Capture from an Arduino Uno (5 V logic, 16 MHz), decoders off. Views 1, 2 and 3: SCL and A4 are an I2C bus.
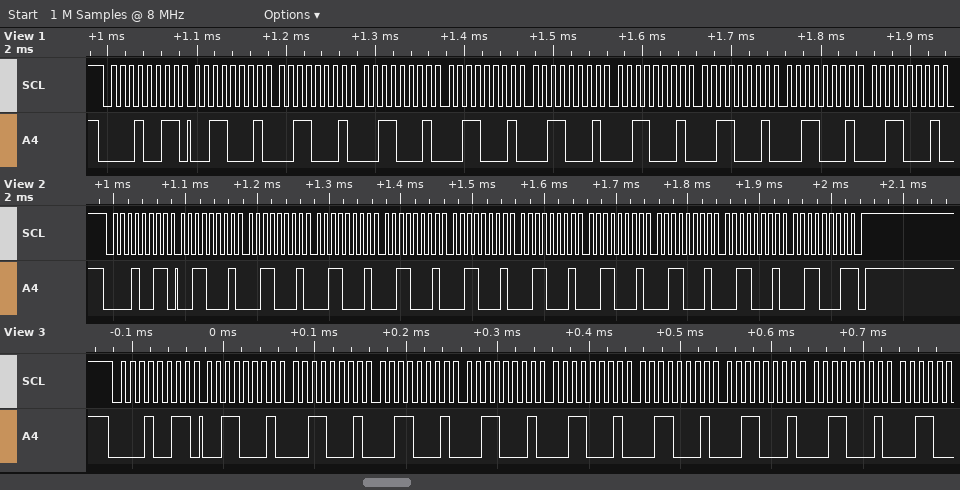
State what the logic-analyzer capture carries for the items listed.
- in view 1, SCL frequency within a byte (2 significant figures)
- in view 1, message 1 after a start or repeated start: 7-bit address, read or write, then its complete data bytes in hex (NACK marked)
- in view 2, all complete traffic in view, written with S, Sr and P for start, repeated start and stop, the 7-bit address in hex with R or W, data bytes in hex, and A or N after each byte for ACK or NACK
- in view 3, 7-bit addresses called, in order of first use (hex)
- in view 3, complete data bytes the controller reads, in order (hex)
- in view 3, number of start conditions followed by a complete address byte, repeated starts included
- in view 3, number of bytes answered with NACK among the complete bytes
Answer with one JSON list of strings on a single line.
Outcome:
["100 kHz", "0x09 read: 31 31 31 31 31 31 31 31 31", "S 09R A 31 A 31 A 31 A 31 A 31 A 31 A 31 A 31 A 31 A 31 N P", "0x09", "31 31 31 31 31 31 31 31", "1", "0"]
